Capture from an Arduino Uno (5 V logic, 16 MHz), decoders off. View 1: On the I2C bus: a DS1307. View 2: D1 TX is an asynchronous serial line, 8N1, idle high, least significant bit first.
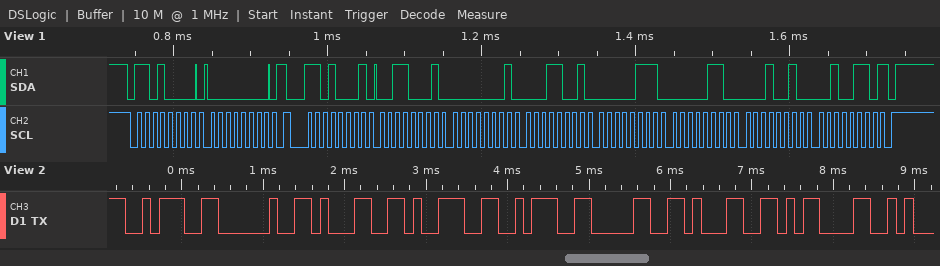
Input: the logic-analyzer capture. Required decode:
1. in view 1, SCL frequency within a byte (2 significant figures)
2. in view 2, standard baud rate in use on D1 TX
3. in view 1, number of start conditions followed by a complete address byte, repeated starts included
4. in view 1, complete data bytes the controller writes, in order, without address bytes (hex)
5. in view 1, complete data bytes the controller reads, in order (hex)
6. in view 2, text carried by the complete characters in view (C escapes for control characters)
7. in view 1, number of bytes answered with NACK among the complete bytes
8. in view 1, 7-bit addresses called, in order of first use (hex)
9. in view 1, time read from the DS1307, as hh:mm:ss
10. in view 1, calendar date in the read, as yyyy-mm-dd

100 kHz
9600 baud
2
00
31 01 19 07 06 12 26
": 19:01\r"
1
0x68
19:01:31
2026-12-06
